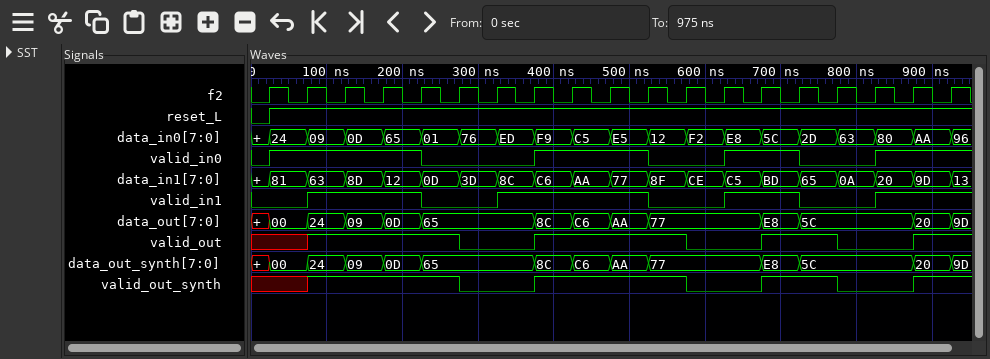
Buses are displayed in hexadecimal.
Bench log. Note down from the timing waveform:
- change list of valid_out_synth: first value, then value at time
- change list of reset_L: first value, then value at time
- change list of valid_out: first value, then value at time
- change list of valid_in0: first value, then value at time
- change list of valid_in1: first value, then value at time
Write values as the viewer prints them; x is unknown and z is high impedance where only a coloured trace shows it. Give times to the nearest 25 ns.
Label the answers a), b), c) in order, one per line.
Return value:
a) x, 1 at 75 ns, 0 at 275 ns, 1 at 375 ns, 0 at 575 ns, 1 at 675 ns, 0 at 775 ns, 1 at 875 ns
b) 0, 1 at 25 ns
c) x, 1 at 75 ns, 0 at 275 ns, 1 at 375 ns, 0 at 575 ns, 1 at 675 ns, 0 at 775 ns, 1 at 875 ns
d) 0, 1 at 25 ns, 0 at 225 ns, 1 at 375 ns, 0 at 525 ns, 1 at 625 ns, 0 at 725 ns, 1 at 825 ns
e) 0, 1 at 75 ns, 0 at 225 ns, 1 at 325 ns, 0 at 525 ns, 1 at 625 ns, 0 at 725 ns, 1 at 825 ns
